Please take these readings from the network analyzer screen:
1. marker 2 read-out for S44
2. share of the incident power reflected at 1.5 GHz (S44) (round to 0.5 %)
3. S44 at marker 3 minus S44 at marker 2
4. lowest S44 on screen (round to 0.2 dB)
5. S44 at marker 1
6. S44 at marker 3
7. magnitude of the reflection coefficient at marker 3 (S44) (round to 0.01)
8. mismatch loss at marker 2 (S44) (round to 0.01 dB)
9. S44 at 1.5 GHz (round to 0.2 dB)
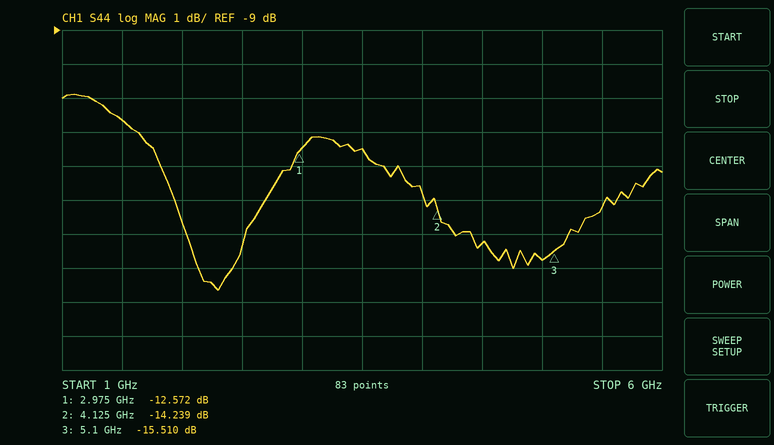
-14.239 dB
7.0 %
-1.271 dB
-16.6 dB
-12.572 dB
-15.510 dB
0.17
0.17 dB
-11.6 dB
